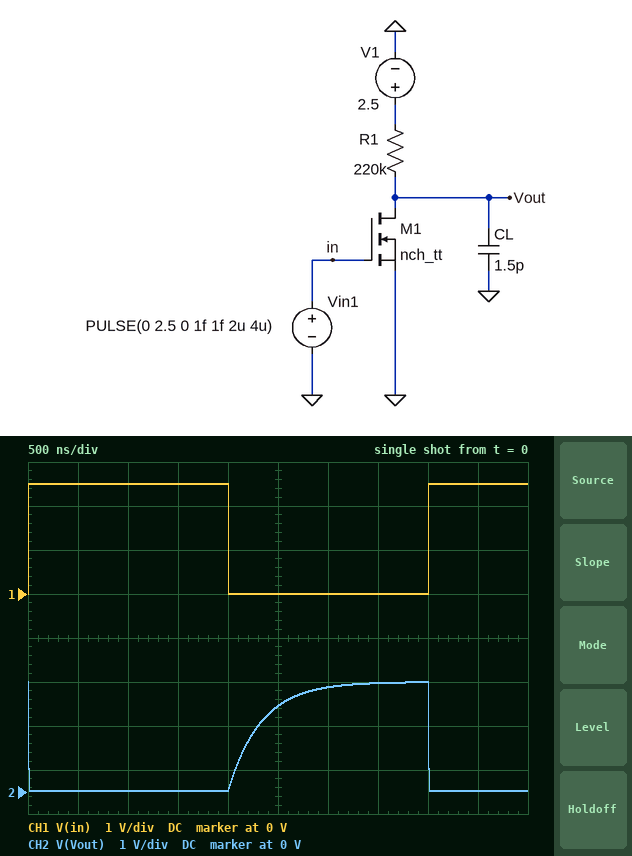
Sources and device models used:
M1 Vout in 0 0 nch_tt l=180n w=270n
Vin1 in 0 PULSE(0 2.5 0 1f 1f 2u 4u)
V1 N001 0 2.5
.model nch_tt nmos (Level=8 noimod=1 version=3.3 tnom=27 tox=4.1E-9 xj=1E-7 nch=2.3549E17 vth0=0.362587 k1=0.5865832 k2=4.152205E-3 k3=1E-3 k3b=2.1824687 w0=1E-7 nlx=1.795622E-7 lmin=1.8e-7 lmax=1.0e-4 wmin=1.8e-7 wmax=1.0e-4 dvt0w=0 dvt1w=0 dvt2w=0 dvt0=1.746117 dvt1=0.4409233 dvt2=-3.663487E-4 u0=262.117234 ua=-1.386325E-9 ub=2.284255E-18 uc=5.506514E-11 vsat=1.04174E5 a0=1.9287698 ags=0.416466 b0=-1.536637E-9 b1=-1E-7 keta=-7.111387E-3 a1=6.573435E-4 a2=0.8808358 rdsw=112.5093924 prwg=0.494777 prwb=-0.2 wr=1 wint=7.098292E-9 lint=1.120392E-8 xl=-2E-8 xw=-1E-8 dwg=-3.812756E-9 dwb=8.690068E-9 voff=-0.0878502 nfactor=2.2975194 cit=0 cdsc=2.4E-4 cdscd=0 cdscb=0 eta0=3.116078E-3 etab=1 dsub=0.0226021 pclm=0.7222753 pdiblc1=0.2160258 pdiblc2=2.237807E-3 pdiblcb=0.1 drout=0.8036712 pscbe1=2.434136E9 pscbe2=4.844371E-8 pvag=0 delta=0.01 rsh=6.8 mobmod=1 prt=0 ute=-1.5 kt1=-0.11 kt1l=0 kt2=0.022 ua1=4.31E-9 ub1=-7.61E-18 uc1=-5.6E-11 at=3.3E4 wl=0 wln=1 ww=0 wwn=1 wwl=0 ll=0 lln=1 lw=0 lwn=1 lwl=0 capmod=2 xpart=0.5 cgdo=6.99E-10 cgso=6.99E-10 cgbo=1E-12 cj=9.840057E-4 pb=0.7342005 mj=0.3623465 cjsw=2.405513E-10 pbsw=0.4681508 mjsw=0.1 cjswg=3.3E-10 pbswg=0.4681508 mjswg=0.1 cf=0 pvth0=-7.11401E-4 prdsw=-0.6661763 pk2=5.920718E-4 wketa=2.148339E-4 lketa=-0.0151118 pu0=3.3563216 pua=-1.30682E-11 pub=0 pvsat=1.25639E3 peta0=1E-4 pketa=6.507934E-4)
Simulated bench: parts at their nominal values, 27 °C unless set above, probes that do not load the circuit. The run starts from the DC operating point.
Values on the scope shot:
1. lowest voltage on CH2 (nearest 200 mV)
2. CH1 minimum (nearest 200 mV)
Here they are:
0 V
0 V
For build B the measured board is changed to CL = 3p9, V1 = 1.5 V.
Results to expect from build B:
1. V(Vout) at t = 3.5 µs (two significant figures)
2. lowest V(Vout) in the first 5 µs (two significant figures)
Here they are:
1.2 V
11 mV
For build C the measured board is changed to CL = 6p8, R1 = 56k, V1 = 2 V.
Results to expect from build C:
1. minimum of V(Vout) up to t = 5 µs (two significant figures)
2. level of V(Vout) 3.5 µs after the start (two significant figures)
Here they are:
56 mV
2.0 V
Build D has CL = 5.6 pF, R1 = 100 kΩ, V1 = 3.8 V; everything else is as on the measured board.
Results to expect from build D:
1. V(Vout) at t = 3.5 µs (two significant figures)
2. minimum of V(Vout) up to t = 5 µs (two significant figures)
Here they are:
3.5 V
61 mV
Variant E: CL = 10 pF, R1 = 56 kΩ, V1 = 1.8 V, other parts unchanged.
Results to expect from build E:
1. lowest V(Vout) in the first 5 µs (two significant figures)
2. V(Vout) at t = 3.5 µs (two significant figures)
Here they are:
50 mV
1.7 V
